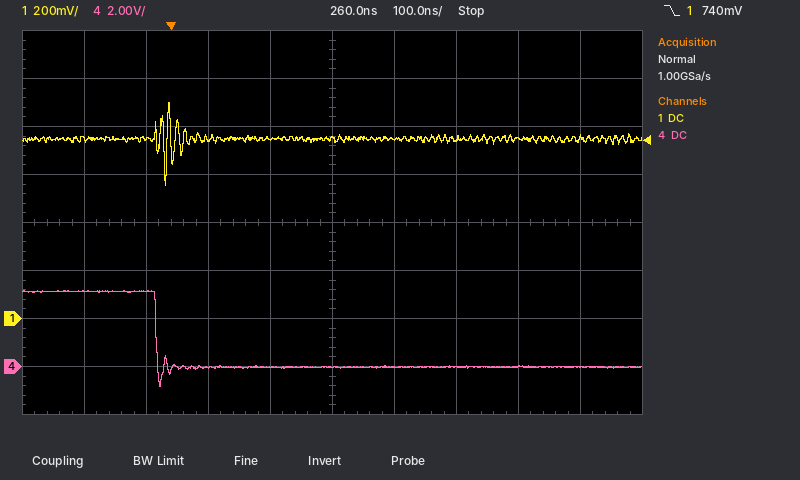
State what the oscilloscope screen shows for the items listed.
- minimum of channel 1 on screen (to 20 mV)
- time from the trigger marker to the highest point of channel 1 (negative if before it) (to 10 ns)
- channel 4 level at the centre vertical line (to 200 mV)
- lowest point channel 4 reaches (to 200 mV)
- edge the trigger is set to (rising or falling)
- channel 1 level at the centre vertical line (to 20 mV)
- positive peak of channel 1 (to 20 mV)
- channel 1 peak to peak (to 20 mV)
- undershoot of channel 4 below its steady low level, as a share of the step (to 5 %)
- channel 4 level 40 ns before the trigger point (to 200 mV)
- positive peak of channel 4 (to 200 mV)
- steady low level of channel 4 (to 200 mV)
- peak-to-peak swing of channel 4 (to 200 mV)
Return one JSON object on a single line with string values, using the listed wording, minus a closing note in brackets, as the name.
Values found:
{"minimum of channel 1 on screen": "560 mV", "time from the trigger marker to the highest point of channel 1 (negative if before it)": "0 ns", "channel 4 level at the centre vertical line": "0.0 V", "lowest point channel 4 reaches": "-800 mV", "edge the trigger is set to": "falling", "channel 1 level at the centre vertical line": "740 mV", "positive peak of channel 1": "900 mV", "channel 1 peak to peak": "340 mV", "undershoot of channel 4 below its steady low level, as a share of the step": "25 %", "channel 4 level 40 ns before the trigger point": "3.2 V", "positive peak of channel 4": "3.2 V", "steady low level of channel 4": "0.0 V", "peak-to-peak swing of channel 4": "4.0 V"}
